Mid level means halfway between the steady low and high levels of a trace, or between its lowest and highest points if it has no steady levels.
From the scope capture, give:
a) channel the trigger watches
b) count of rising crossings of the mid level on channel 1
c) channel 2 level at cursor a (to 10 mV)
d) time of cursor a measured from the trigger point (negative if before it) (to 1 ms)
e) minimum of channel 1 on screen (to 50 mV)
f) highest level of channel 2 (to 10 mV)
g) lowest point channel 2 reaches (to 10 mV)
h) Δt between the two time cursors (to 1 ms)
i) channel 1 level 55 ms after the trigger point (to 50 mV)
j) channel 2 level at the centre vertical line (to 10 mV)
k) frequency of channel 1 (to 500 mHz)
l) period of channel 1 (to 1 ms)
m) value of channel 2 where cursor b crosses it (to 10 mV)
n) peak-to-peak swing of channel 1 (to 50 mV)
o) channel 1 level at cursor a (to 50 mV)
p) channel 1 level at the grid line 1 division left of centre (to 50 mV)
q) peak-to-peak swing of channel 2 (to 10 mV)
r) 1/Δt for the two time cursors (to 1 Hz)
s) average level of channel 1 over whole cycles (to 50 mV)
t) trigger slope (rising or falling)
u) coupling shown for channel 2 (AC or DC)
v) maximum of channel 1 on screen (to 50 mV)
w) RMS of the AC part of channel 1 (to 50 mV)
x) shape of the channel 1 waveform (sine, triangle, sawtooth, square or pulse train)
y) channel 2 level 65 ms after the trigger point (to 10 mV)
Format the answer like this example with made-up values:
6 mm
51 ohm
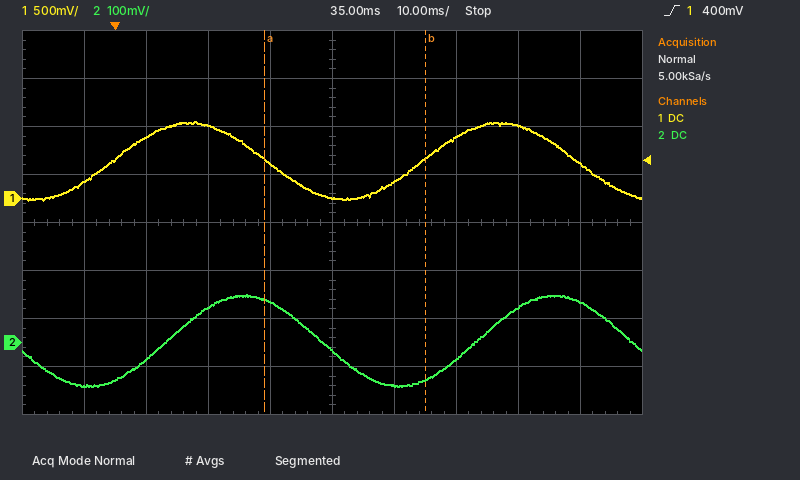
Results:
channel 1
2
90 mV
+24 ms
0 mV
100 mV
-90 mV
26 ms
650 mV
-20 mV
20.0 Hz
50 ms
-80 mV
800 mV
400 mV
350 mV
190 mV
38 Hz
400 mV
rising
DC
800 mV
300 mV
sine
70 mV
